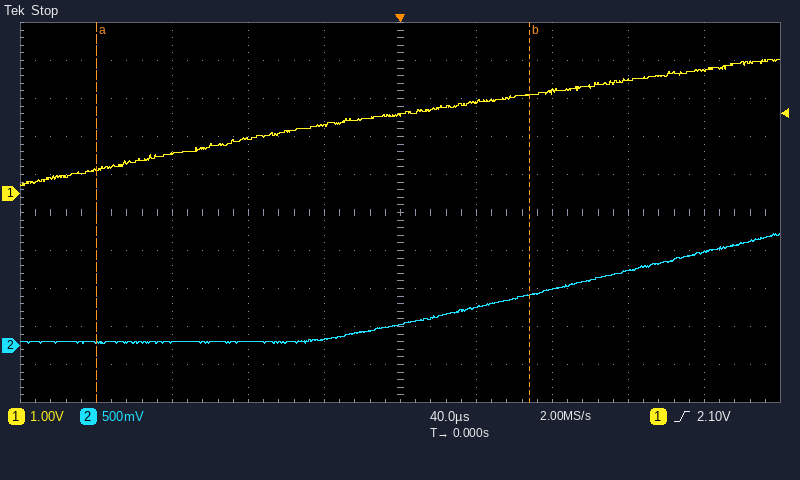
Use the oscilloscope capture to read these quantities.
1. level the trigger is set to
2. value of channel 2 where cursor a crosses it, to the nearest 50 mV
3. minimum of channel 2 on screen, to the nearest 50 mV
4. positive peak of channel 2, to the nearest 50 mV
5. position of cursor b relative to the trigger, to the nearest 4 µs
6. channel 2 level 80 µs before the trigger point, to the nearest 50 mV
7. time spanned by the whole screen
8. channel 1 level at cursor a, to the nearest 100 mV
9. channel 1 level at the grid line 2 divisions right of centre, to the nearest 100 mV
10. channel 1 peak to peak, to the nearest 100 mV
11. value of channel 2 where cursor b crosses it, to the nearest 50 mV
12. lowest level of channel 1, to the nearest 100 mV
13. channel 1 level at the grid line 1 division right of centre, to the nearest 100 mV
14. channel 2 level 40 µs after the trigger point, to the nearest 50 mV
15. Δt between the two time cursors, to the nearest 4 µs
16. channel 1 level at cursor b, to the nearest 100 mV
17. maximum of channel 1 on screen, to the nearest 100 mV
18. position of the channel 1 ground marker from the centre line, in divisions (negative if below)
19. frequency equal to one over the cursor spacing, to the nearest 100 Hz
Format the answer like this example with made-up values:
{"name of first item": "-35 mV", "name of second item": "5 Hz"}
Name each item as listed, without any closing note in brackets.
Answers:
{"level the trigger is set to": "2.10 V", "value of channel 2 where cursor a crosses it, to the nearest 50 mV": "50 mV", "minimum of channel 2 on screen, to the nearest 50 mV": "50 mV", "positive peak of channel 2, to the nearest 50 mV": "1.45 V", "position of cursor b relative to the trigger, to the nearest 4 µs": "+68 µs", "channel 2 level 80 µs before the trigger point, to the nearest 50 mV": "50 mV", "time spanned by the whole screen": "400 µs", "channel 1 level at cursor a, to the nearest 100 mV": "600 mV", "channel 1 level at the grid line 2 divisions right of centre, to the nearest 100 mV": "2.7 V", "channel 1 peak to peak, to the nearest 100 mV": "3.3 V", "value of channel 2 where cursor b crosses it, to the nearest 50 mV": "650 mV", "lowest level of channel 1, to the nearest 100 mV": "200 mV", "channel 1 level at the grid line 1 division right of centre, to the nearest 100 mV": "2.4 V", "channel 2 level 40 µs after the trigger point, to the nearest 50 mV": "500 mV", "Δt between the two time cursors, to the nearest 4 µs": "228 µs", "channel 1 level at cursor b, to the nearest 100 mV": "2.6 V", "maximum of channel 1 on screen, to the nearest 100 mV": "3.5 V", "position of the channel 1 ground marker from the centre line, in divisions": "+0.5 div", "frequency equal to one over the cursor spacing, to the nearest 100 Hz": "4.4 kHz"}
